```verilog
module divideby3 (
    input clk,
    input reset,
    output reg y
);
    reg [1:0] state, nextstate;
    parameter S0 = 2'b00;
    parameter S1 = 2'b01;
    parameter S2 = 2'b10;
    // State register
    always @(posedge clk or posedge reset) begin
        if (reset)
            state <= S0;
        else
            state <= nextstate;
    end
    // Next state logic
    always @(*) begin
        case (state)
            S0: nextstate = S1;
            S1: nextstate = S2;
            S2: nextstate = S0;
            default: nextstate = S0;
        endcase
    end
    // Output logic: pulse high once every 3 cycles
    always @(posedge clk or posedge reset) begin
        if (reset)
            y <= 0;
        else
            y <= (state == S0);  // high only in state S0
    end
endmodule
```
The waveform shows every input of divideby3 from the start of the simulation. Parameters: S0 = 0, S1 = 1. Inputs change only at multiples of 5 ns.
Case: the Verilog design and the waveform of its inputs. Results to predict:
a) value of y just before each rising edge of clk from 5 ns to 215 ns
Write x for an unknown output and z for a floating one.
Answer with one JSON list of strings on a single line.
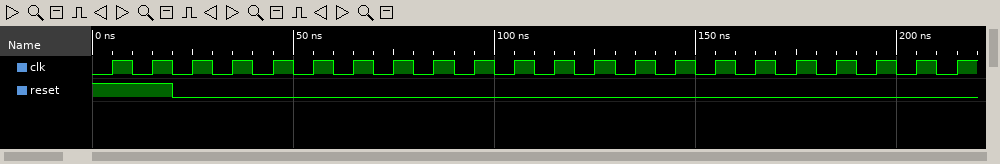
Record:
["0 0 0 1 0 0 1 0 0 1 0 0 1 0 0 1 0 0 1 0 0 1"]
